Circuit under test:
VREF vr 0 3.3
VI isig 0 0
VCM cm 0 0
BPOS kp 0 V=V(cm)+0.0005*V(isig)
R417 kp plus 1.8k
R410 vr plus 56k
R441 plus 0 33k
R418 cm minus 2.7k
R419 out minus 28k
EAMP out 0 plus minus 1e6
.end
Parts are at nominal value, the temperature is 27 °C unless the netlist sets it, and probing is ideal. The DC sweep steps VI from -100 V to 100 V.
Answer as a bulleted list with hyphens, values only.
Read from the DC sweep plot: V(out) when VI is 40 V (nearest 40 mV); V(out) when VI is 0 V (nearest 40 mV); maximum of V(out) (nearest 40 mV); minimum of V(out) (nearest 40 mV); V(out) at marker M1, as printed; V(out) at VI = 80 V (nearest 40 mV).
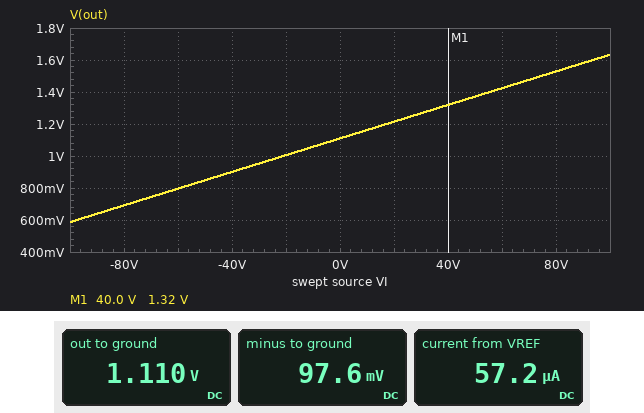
- 1.32 V
- 1.12 V
- 1.64 V
- 600 mV
- 1.32 V
- 1.52 V
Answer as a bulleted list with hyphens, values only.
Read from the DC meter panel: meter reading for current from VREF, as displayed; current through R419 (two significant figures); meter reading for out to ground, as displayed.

- 57.2 µA
- 36 µA
- 1.110 V
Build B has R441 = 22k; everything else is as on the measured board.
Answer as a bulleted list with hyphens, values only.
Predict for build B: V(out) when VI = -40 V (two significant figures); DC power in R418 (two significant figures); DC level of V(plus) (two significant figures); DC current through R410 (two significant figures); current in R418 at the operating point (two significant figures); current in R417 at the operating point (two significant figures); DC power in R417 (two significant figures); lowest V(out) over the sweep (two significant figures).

- 880 mV
- 3.4 µW
- 95 mV
- 57 µA
- 35 µA
- 53 µA
- 5.0 µW
- 570 mV
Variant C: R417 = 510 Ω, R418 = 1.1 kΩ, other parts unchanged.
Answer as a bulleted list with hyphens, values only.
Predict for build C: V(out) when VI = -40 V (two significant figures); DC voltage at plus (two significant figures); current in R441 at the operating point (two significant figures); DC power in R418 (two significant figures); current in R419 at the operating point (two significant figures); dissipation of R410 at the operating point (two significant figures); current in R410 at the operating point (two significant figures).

- 260 mV
- 29 mV
- 890 nA
- 780 nW
- 27 µA
- 190 µW
- 58 µA
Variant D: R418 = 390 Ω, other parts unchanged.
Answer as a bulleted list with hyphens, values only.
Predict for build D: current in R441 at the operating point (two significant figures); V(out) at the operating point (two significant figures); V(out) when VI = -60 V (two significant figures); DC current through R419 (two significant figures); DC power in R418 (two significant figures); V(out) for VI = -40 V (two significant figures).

- 3.0 µA
- 7.1 V
- 5.1 V
- 250 µA
- 24 µW
- 5.8 V
